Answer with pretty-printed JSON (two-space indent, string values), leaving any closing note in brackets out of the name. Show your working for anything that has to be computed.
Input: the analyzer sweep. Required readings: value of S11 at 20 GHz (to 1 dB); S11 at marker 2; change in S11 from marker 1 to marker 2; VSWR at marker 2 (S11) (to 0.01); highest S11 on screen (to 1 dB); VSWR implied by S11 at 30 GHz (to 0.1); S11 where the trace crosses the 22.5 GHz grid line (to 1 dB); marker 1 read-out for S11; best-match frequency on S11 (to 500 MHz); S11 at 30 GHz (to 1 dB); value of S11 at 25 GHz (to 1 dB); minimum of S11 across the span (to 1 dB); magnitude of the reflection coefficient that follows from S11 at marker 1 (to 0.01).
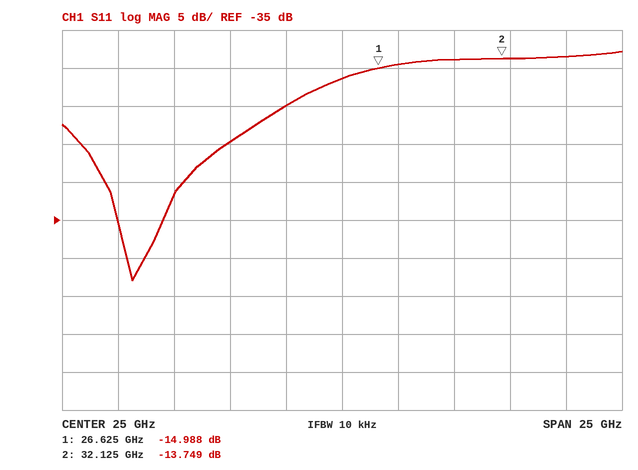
{
  "value of S11 at 20 GHz": "-25 dB",
  "S11 at marker 2": "-13.749 dB",
  "change in S11 from marker 1 to marker 2": "-13.749 − (-14.988) = 1.239 dB",
  "VSWR at marker 2 (S11)": "(1 + 0.2054)/(1 − 0.2054) ≈ 1.52",
  "highest S11 on screen": "-13 dB",
  "VSWR implied by S11 at 30 GHz": "|Γ| = 10^(-14/20) = 0.1995; VSWR = (1 + 0.1995)/(1 − 0.1995) ≈ 1.5",
  "S11 where the trace crosses the 22.5 GHz grid line": "-20 dB",
  "marker 1 read-out for S11": "-14.988 dB",
  "best-match frequency on S11": "15.5 GHz",
  "S11 at 30 GHz": "-14 dB",
  "value of S11 at 25 GHz": "-16 dB",
  "minimum of S11 across the span": "-43 dB",
  "magnitude of the reflection coefficient that follows from S11 at marker 1": "10^(-14.988/20) ≈ 0.18"
}
